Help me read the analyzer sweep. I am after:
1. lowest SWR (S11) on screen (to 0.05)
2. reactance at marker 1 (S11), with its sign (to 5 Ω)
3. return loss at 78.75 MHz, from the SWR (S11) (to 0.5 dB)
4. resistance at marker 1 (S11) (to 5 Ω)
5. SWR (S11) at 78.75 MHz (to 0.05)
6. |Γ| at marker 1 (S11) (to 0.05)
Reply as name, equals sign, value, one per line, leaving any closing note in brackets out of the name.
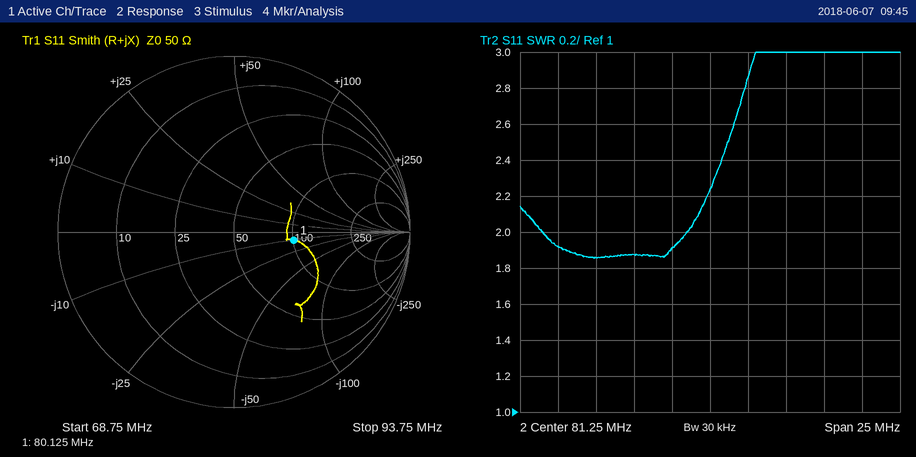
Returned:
lowest SWR (S11) on screen = 1.85
reactance at marker 1 (S11), with its sign = -10 Ω
return loss at 78.75 MHz, from the SWR (S11) = 10.0 dB
resistance at marker 1 (S11) = 100 Ω
SWR (S11) at 78.75 MHz = 1.90
|Γ| at marker 1 (S11) = 0.35
